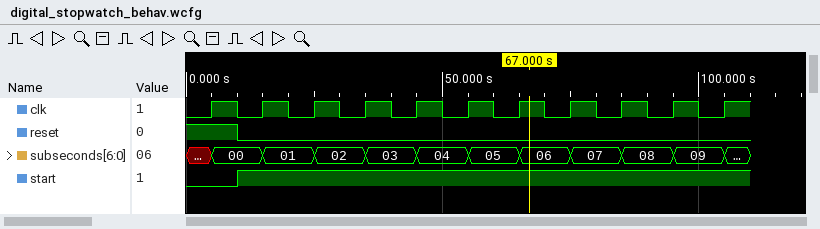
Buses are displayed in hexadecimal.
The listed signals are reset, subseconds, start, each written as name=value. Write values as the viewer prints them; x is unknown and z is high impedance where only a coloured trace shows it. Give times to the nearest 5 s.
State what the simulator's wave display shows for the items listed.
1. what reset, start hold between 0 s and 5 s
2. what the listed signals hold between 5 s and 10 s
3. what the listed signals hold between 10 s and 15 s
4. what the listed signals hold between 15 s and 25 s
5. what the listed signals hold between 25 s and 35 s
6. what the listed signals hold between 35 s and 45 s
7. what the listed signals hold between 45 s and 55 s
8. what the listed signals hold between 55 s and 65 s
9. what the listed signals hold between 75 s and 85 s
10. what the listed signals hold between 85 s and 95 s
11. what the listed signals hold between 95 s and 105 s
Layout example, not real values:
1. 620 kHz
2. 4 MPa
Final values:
1. reset=1, start=0
2. reset=1, subseconds=00, start=0
3. reset=0, subseconds=00, start=1
4. reset=0, subseconds=01, start=1
5. reset=0, subseconds=02, start=1
6. reset=0, subseconds=03, start=1
7. reset=0, subseconds=04, start=1
8. reset=0, subseconds=05, start=1
9. reset=0, subseconds=07, start=1
10. reset=0, subseconds=08, start=1
11. reset=0, subseconds=09, start=1
